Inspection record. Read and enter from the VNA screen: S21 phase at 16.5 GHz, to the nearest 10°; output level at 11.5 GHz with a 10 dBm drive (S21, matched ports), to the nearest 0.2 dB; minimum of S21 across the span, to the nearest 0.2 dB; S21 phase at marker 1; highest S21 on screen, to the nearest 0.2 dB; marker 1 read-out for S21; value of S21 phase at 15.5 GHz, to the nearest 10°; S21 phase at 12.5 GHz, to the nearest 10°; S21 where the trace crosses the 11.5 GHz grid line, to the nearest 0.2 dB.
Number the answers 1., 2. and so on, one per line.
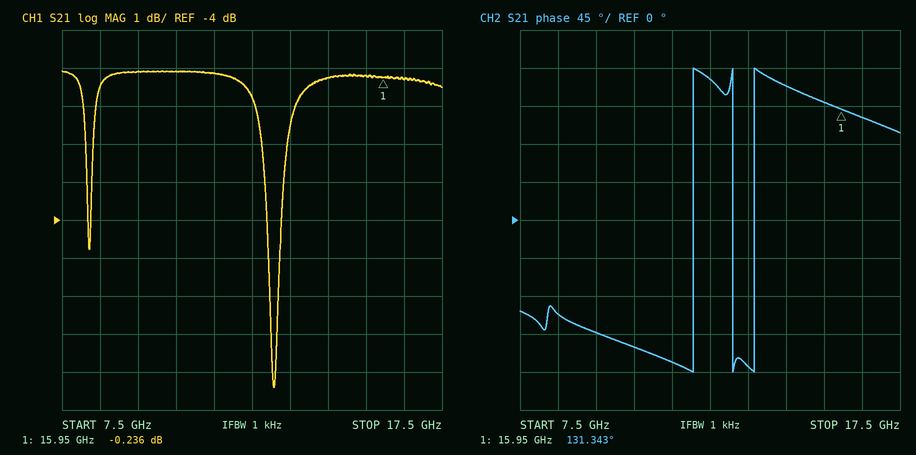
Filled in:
1. 120°
2. 9.8 dBm
3. -8.4 dB
4. 131.343°
5. 0.0 dB
6. -0.236 dB
7. 140°
8. 170°
9. -0.2 dB
